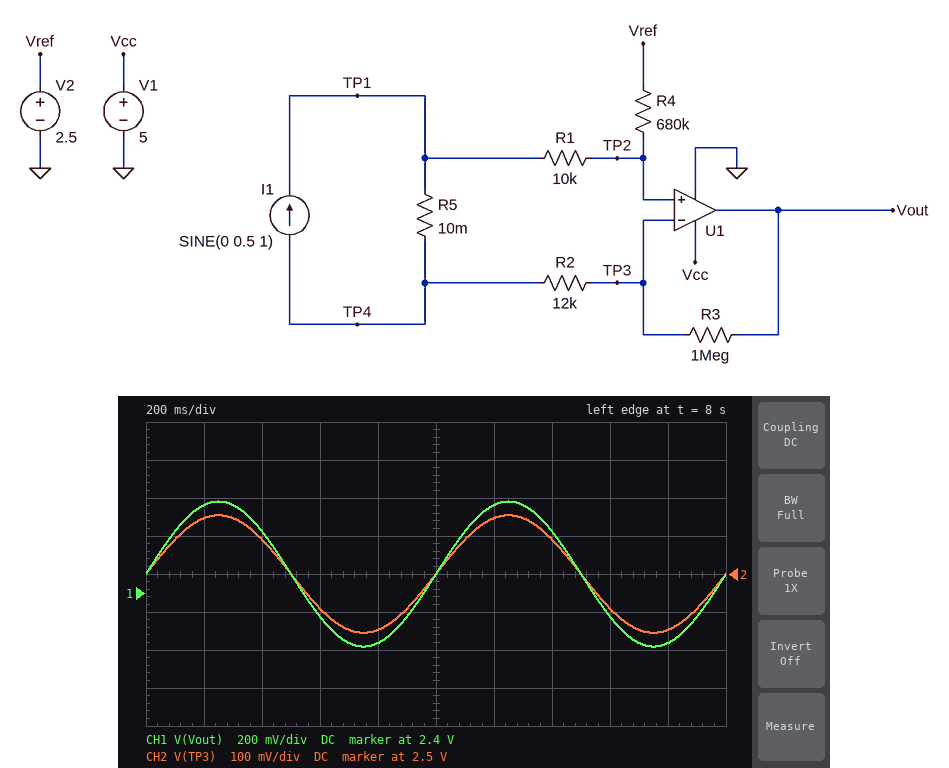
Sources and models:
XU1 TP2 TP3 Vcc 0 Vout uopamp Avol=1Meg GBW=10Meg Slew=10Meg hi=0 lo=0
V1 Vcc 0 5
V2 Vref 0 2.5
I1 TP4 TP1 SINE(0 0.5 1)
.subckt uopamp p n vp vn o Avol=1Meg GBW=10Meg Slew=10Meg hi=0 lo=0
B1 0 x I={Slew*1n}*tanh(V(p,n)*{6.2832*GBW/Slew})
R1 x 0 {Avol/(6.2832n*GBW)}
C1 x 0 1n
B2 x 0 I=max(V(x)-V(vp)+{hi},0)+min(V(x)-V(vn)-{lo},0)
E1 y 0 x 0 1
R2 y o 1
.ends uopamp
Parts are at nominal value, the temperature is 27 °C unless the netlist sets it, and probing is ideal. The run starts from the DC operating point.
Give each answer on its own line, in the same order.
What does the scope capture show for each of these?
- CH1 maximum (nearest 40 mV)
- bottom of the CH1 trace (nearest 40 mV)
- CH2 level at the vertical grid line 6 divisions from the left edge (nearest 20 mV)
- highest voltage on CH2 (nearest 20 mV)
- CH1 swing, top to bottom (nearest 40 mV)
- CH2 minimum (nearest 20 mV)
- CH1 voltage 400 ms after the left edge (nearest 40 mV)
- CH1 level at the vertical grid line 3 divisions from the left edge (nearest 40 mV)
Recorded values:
2.88 V
2.12 V
2.64 V
2.66 V
760 mV
2.34 V
2.72 V
2.28 V
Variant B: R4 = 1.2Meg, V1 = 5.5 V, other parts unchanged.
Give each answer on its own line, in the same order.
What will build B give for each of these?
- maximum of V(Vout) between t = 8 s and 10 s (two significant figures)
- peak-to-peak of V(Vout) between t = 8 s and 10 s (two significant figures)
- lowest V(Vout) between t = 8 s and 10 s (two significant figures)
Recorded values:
3.0 V
1.0 V
2.0 V
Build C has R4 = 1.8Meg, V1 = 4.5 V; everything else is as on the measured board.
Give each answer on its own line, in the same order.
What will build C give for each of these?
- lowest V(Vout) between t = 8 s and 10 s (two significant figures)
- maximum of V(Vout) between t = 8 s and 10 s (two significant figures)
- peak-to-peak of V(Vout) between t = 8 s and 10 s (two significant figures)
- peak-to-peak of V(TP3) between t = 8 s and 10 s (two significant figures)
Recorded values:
1.9 V
3.1 V
1.3 V
820 mV
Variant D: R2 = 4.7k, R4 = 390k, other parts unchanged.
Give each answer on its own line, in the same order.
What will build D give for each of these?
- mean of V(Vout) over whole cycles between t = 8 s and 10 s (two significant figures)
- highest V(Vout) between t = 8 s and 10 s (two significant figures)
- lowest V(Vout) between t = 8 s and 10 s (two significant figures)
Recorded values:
2.5 V
3.0 V
2.0 V
